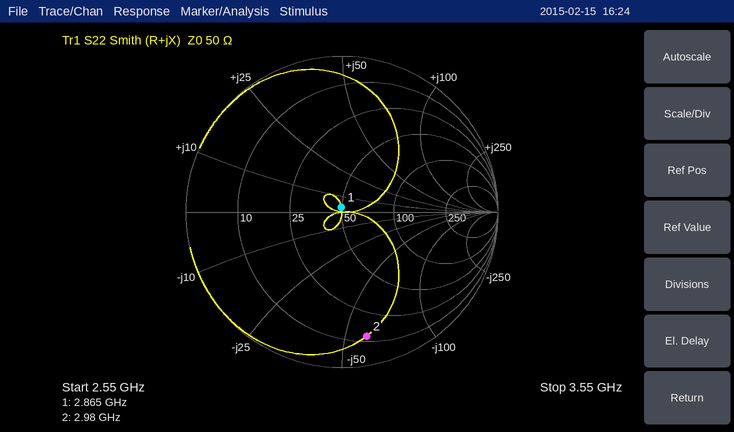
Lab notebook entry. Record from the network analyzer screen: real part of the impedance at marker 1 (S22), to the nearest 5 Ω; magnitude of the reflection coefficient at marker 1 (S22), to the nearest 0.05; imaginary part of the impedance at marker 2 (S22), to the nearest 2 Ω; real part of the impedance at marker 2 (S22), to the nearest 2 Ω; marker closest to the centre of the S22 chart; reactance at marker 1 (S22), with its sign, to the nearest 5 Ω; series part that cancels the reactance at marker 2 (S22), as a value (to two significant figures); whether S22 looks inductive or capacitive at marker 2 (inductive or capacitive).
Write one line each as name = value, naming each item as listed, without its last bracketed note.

real part of the impedance at marker 1 (S22), to the nearest 5 Ω = 50 Ω
magnitude of the reflection coefficient at marker 1 (S22), to the nearest 0.05 = 0.05
imaginary part of the impedance at marker 2 (S22), to the nearest 2 Ω = -60 Ω
real part of the impedance at marker 2 (S22), to the nearest 2 Ω = 12 Ω
marker closest to the centre of the S22 chart = marker 1
reactance at marker 1 (S22), with its sign, to the nearest 5 Ω = +5 Ω
series part that cancels the reactance at marker 2 (S22), as a value = 3.2 nH
whether S22 looks inductive or capacitive at marker 2 = capacitive
